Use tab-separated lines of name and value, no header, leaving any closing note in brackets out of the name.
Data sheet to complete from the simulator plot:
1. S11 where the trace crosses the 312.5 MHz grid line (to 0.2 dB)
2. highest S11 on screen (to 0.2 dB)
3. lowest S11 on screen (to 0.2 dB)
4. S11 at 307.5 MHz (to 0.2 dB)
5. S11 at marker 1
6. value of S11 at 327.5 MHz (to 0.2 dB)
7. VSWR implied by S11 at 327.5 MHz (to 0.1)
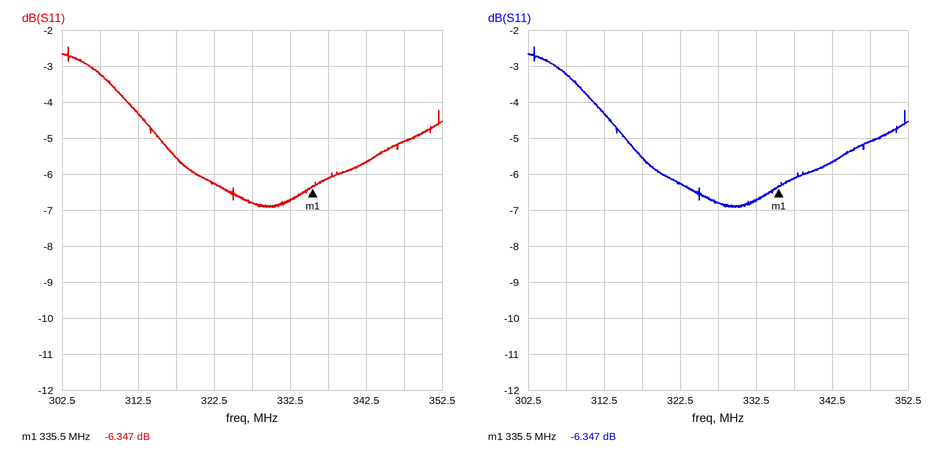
S11 where the trace crosses the 312.5 MHz grid line	-4.4 dB
highest S11 on screen	-2.4 dB
lowest S11 on screen	-7.0 dB
S11 at 307.5 MHz	-3.2 dB
S11 at marker 1	-6.347 dB
value of S11 at 327.5 MHz	-6.8 dB
VSWR implied by S11 at 327.5 MHz	2.7
